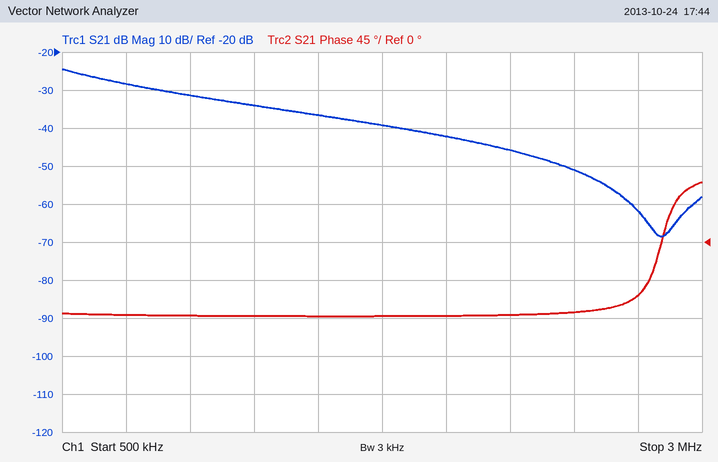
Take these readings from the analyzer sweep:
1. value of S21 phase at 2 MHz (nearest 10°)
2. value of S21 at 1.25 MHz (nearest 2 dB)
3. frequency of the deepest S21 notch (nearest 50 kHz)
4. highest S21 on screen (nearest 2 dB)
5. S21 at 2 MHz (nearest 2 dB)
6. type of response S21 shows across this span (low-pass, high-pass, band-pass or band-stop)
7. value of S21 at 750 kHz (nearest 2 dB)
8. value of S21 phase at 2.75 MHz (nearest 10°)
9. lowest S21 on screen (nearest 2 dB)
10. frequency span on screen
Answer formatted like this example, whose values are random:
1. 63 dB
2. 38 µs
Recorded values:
1. -90°
2. -34 dB
3. 2.85 MHz
4. -24 dB
5. -42 dB
6. low-pass
7. -28 dB
8. -60°
9. -68 dB
10. 2.5 MHz
